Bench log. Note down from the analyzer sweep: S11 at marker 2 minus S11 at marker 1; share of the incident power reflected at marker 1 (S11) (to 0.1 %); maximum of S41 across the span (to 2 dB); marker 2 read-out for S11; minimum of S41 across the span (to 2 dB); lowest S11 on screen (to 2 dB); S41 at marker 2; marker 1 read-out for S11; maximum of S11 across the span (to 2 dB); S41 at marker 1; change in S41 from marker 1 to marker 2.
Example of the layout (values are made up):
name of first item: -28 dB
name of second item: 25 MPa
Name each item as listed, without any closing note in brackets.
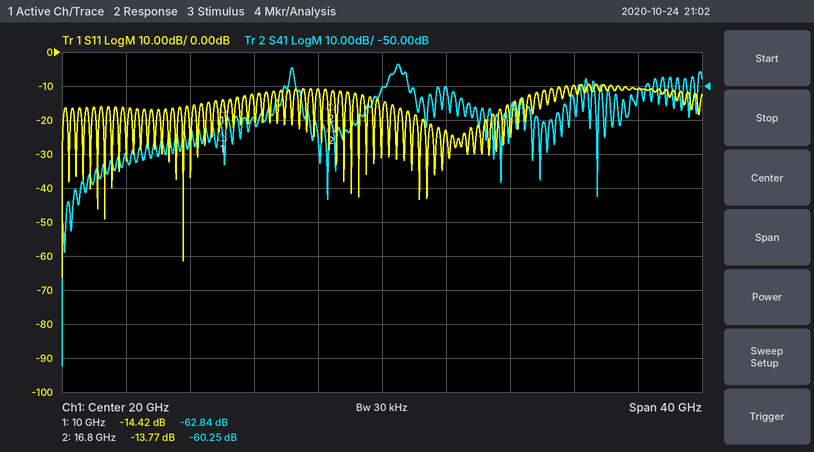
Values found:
S11 at marker 2 minus S11 at marker 1: 0.65 dB
share of the incident power reflected at marker 1 (S11): 3.6 %
maximum of S41 across the span: -44 dB
marker 2 read-out for S11: -13.77 dB
minimum of S41 across the span: -132 dB
lowest S11 on screen: -66 dB
S41 at marker 2: -60.25 dB
marker 1 read-out for S11: -14.42 dB
maximum of S11 across the span: -10 dB
S41 at marker 1: -62.84 dB
change in S41 from marker 1 to marker 2: 2.59 dB
